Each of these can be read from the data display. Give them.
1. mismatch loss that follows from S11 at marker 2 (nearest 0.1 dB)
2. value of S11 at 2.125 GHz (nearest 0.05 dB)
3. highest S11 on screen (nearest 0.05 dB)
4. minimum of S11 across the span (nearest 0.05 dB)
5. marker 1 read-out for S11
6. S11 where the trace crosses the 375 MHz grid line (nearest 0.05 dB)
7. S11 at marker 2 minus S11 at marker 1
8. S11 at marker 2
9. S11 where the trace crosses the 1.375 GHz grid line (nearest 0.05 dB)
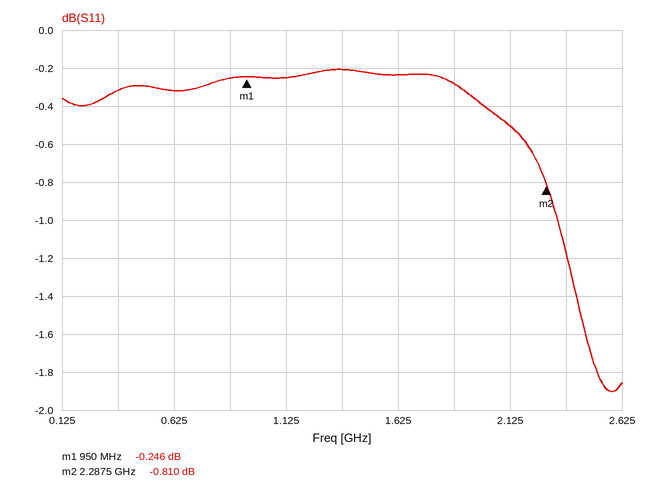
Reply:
7.7 dB
-0.50 dB
-0.20 dB
-1.90 dB
-0.246 dB
-0.30 dB
-0.564 dB
-0.810 dB
-0.20 dB
